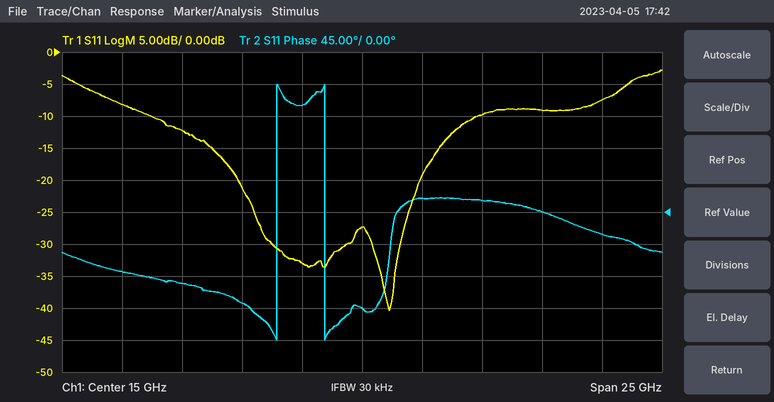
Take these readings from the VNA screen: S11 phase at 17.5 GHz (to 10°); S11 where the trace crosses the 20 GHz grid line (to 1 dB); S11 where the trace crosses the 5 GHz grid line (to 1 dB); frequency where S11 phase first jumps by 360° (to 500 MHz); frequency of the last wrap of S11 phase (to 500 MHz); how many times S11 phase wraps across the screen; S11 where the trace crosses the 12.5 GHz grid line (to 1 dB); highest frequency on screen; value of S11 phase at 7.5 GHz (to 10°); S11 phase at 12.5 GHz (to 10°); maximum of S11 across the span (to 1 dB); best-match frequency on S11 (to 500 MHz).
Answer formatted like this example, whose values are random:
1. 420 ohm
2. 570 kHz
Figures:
1. 20°
2. -10 dB
3. -8 dB
4. 11.5 GHz
5. 13.5 GHz
6. 2
7. -33 dB
8. 27.5 GHz
9. -100°
10. 150°
11. -3 dB
12. 16.0 GHz
